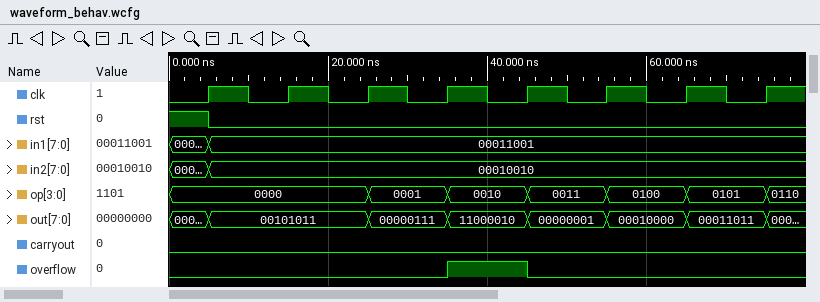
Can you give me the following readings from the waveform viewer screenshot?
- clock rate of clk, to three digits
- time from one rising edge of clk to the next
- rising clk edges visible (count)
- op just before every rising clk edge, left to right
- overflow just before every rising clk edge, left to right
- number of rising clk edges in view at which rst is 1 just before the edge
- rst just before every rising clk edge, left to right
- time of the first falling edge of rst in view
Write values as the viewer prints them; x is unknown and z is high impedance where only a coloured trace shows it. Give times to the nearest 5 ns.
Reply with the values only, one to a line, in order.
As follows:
100 MHz
10 ns
8
0000, 0000, 0000, 0001, 0010, 0011, 0100, 0101
0 0 0 0 1 0 0 0
1
1 0 0 0 0 0 0 0
5 ns
